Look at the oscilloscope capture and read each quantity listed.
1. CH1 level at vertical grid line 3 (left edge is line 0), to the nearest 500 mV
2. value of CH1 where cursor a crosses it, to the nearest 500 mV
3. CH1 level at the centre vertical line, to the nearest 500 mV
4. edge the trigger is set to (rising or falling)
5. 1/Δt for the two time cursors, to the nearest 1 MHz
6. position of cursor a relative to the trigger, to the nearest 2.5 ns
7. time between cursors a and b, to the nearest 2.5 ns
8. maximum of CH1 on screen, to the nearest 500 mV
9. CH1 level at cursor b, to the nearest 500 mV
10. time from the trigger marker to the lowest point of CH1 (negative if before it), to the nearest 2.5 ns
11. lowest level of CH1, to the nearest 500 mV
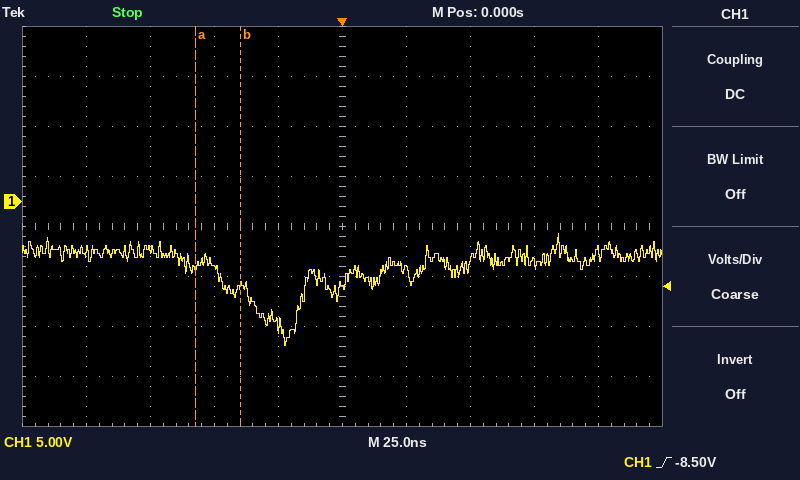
-6.5 V
-6.5 V
-8.5 V
rising
57 MHz
-57.5 ns
17.5 ns
-3.0 V
-8.5 V
-22.5 ns
-14.5 V
